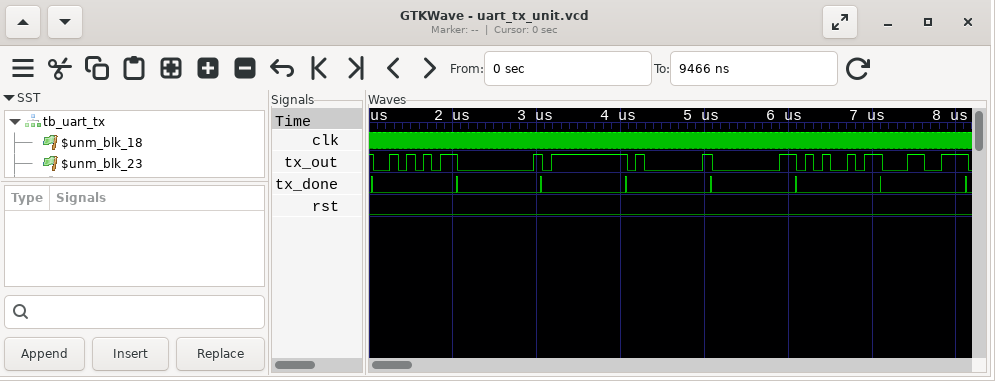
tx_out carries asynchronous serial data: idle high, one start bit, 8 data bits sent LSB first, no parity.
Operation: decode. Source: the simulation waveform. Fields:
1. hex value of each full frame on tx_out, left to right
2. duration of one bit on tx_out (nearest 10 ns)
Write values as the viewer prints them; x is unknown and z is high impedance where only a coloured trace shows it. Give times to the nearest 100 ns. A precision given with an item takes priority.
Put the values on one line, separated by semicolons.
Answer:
AA, 00, FF, 01, 80, A5, CC; 100 ns
